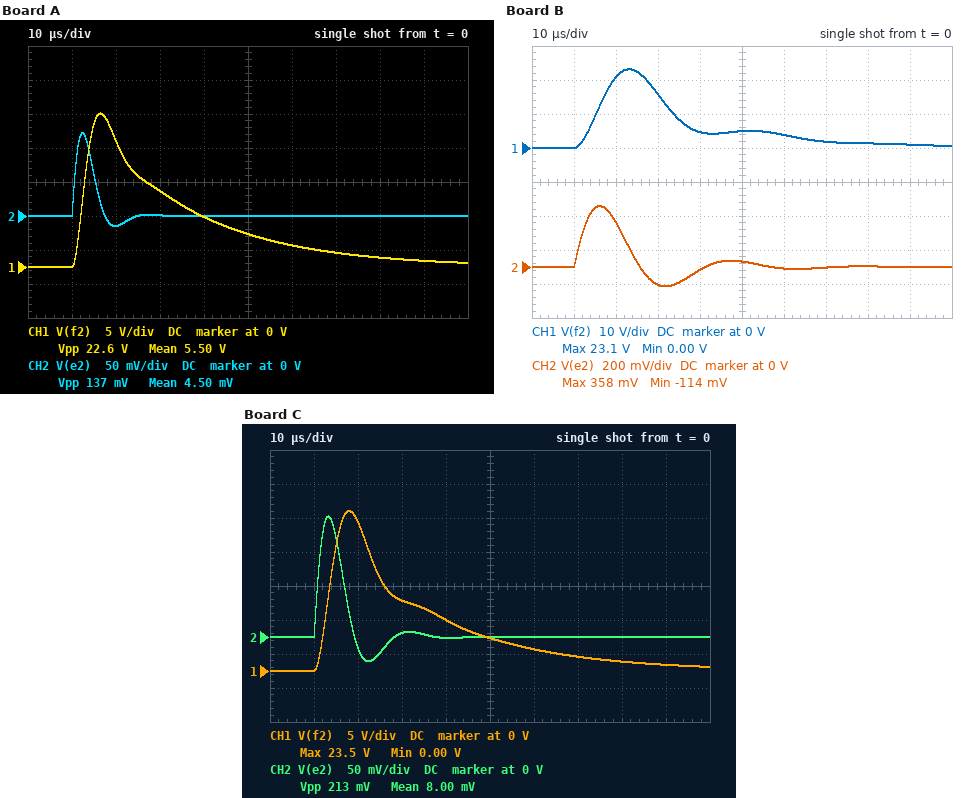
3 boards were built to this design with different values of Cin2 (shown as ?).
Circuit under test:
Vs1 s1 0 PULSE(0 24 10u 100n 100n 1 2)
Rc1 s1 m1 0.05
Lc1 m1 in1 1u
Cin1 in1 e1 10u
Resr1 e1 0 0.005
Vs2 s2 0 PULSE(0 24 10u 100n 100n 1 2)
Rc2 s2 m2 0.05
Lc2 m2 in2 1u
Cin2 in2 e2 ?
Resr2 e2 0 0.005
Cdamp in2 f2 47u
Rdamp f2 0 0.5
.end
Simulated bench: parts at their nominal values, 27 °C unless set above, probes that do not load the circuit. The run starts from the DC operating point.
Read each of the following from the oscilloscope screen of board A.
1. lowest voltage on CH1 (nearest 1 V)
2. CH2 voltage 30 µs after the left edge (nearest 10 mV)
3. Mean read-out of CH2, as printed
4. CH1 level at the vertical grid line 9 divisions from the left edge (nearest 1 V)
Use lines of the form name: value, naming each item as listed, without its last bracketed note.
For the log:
lowest voltage on CH1: 0 V
CH2 voltage 30 µs after the left edge: 0 V
Mean read-out of CH2, as printed: 4.50 mV
CH1 level at the vertical grid line 9 divisions from the left edge: 1 V
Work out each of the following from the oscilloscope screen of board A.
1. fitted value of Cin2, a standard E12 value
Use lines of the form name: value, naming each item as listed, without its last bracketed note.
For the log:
fitted value of Cin2, a standard E12 value: 3.9 µF
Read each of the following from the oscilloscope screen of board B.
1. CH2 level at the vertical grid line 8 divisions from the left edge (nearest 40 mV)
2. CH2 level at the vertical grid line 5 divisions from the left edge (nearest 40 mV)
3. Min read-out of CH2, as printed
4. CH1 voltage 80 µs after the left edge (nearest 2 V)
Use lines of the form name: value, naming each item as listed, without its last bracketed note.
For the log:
CH2 level at the vertical grid line 8 divisions from the left edge: 0 V
CH2 level at the vertical grid line 5 divisions from the left edge: 40 mV
Min read-out of CH2, as printed: -114 mV
CH1 voltage 80 µs after the left edge: 2 V
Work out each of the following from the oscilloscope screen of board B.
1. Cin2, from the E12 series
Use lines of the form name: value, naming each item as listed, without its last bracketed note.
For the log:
Cin2, from the E12 series: 22 µF
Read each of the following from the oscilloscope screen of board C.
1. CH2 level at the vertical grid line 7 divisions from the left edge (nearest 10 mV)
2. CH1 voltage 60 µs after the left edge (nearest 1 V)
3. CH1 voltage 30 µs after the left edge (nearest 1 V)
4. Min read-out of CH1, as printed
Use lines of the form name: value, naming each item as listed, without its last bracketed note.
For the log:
CH2 level at the vertical grid line 7 divisions from the left edge: 0 V
CH1 voltage 60 µs after the left edge: 3 V
CH1 voltage 30 µs after the left edge: 10 V
Min read-out of CH1, as printed: 0.00 V
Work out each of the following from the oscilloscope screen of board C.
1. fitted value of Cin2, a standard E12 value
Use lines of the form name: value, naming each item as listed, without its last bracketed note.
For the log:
fitted value of Cin2, a standard E12 value: 6.8 µF
